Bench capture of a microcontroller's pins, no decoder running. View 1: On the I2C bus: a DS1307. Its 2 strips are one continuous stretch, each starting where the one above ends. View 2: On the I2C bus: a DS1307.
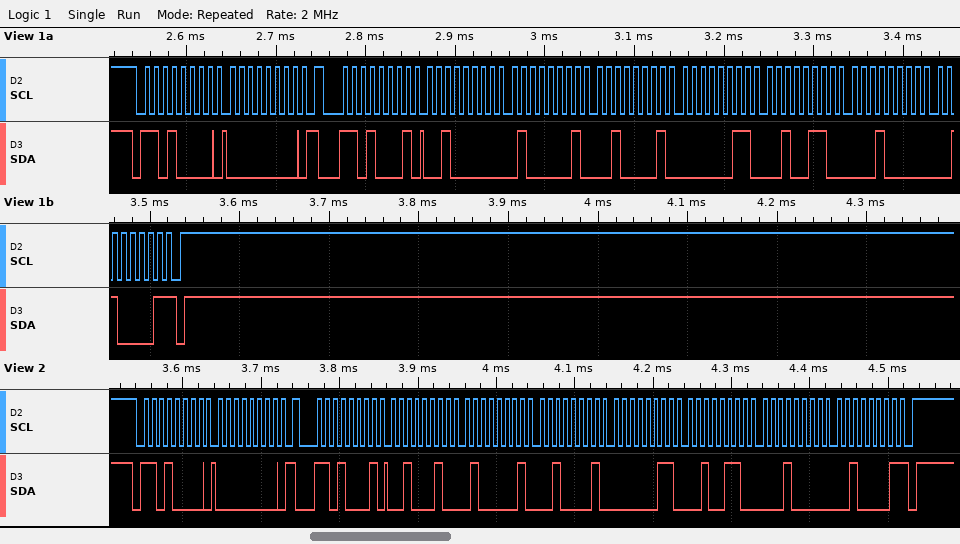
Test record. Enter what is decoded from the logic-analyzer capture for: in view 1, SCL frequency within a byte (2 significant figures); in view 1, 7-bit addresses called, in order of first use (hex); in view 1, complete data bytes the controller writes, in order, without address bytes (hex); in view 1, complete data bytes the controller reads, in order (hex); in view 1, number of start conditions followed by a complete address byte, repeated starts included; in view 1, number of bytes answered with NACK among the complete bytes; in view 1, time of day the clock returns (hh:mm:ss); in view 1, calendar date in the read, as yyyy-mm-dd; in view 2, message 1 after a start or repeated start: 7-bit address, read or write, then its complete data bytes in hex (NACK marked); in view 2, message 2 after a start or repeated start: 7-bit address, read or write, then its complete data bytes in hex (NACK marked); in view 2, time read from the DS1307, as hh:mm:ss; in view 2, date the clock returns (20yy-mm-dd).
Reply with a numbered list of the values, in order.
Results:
1. 100 kHz
2. 0x68
3. 00
4. 20 41 21 03 26 10 21
5. 2
6. 1
7. 21:41:20
8. 2021-10-26
9. 0x68 write: 00
10. 0x68 read: 22 41 21 03 26 10 21 NACK
11. 21:41:22
12. 2021-10-26
